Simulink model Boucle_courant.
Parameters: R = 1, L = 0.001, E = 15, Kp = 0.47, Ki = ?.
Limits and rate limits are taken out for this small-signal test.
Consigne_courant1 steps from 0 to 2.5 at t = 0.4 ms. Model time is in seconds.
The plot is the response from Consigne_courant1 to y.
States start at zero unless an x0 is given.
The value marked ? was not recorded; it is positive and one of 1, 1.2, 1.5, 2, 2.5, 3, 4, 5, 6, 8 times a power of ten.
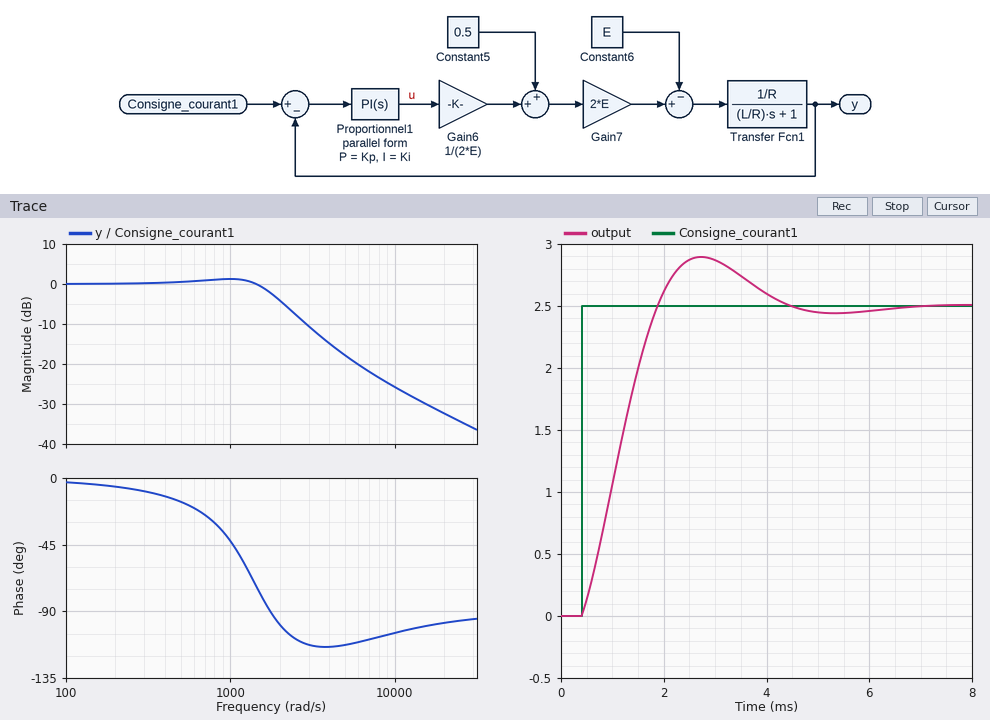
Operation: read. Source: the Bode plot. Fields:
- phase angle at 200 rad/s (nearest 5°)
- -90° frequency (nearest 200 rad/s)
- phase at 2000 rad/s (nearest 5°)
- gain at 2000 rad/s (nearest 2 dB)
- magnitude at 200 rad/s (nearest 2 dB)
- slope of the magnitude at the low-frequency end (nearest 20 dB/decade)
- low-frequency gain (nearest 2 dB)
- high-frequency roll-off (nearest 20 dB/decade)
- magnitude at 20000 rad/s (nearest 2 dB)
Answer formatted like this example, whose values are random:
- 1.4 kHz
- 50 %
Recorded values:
- -5°
- 1800 rad/s
- -100°
- -4 dB
- 0 dB
- 0 dB/decade
- 0 dB
- -20 dB/decade
- -32 dB
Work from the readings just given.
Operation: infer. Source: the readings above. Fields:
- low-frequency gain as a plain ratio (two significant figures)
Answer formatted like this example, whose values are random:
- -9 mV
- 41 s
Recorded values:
- 1.0
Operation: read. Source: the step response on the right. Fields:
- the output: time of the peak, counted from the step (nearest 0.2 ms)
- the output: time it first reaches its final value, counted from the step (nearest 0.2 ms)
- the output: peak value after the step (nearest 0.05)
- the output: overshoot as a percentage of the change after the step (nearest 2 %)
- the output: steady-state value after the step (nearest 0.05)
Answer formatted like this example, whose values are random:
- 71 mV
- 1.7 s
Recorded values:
- 2.4 ms
- 1.4 ms
- 2.90
- 16 %
- 2.50
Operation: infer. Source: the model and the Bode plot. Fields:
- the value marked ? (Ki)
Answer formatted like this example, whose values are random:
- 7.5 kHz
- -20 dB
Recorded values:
- 2000
